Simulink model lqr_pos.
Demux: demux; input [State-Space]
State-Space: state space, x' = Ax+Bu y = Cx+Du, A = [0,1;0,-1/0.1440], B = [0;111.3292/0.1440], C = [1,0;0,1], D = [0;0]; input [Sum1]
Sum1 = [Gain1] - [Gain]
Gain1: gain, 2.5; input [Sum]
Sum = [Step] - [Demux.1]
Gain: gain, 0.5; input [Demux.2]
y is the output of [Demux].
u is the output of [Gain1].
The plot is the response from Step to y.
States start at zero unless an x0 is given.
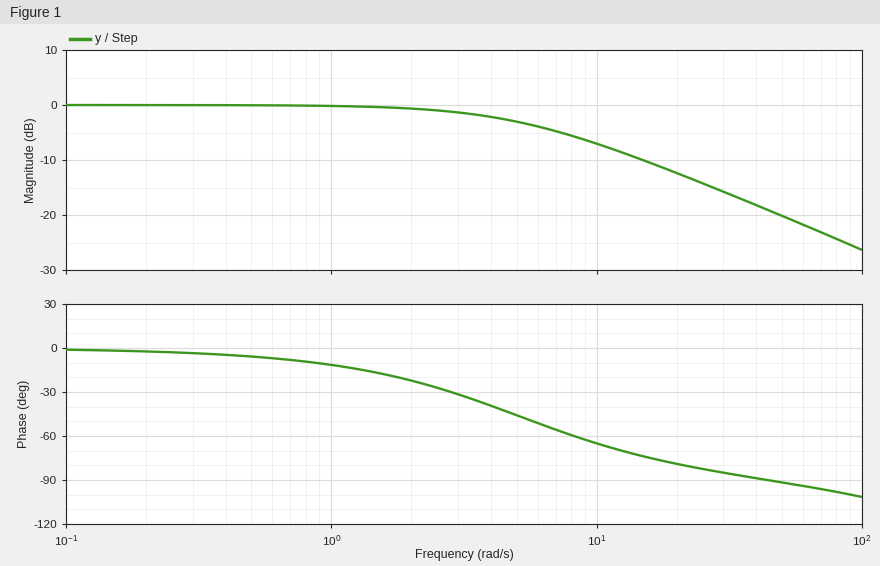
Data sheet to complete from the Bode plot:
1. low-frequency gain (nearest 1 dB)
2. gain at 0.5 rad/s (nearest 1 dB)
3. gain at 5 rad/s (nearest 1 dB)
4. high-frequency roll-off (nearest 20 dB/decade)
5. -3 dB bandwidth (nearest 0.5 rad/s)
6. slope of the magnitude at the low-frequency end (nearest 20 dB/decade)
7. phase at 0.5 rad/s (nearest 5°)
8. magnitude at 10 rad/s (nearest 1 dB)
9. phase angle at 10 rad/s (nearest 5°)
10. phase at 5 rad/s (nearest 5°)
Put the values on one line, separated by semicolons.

0 dB; 0 dB; -3 dB; -20 dB/decade; 5.0 rad/s; 0 dB/decade; -5°; -7 dB; -65°; -45°
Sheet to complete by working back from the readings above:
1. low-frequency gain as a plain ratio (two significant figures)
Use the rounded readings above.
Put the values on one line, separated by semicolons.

1.0
